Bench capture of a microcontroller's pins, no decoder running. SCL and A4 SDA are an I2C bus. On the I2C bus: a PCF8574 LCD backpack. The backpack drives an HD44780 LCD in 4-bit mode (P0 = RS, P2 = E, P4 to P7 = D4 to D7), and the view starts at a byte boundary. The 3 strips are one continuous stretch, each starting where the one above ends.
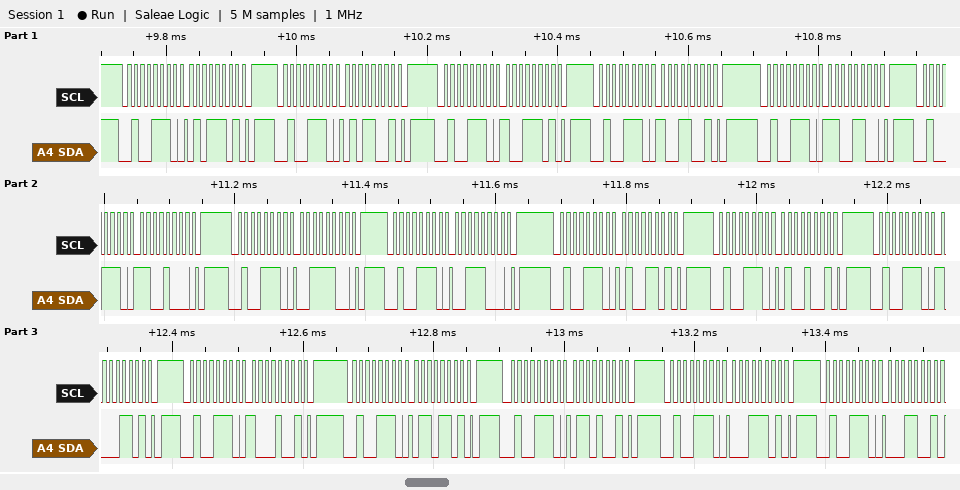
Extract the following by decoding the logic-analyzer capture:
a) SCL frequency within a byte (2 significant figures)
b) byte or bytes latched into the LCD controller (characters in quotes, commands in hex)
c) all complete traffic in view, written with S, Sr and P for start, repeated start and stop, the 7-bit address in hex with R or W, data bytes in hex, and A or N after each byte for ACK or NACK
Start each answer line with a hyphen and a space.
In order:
- 100 kHz
- 'Y' 0xC3 'H' 'a'
- S 27W A 5D A P S 27W A 59 A P S 27W A 9D A P S 27W A 99 A P S 27W A CC A P S 27W A C8 A P S 27W A 3C A P S 27W A 38 A P S 27W A 4D A P S 27W A 49 A P S 27W A 8D A P S 27W A 89 A P S 27W A 6D A P S 27W A 69 A P S 27W A 1D A P S 27W A 19 A
